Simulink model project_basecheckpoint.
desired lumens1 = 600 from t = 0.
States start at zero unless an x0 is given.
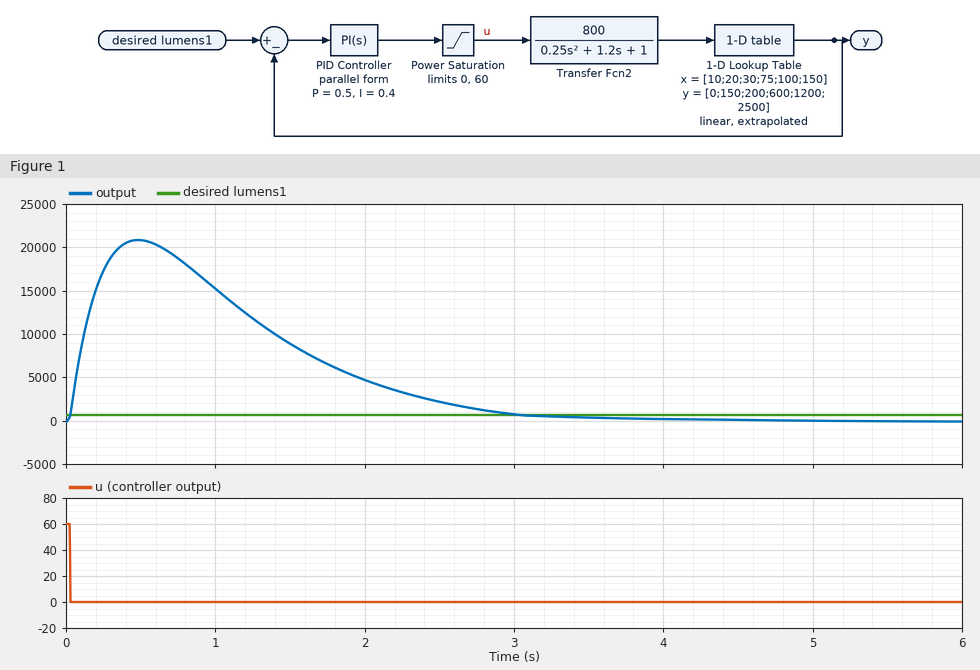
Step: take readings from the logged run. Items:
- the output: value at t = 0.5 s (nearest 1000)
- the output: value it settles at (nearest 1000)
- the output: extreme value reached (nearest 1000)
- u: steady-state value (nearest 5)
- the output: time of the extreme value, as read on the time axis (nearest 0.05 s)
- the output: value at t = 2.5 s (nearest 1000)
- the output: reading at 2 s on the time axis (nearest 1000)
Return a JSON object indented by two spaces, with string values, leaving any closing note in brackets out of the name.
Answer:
{
  "the output: value at t = 0.5 s": "21000",
  "the output: value it settles at": "0",
  "the output: extreme value reached": "21000",
  "u: steady-state value": "0",
  "the output: time of the extreme value, as read on the time axis": "0.50 s",
  "the output: value at t = 2.5 s": "2000",
  "the output: reading at 2 s on the time axis": "5000"
}
